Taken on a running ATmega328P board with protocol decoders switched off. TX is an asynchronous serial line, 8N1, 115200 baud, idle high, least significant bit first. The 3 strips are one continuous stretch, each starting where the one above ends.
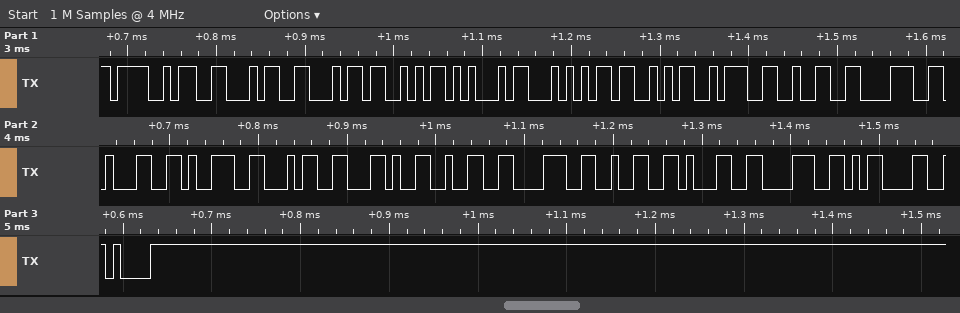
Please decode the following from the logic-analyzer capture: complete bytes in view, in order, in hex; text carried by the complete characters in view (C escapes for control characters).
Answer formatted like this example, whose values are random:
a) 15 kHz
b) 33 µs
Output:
a) 4F 46 46 53 45 54 53 3A 32 38 31 39 34 2C 32 38 32 31 38 0D 0A
b) "OFFSETS:28194,28218\r\n"
